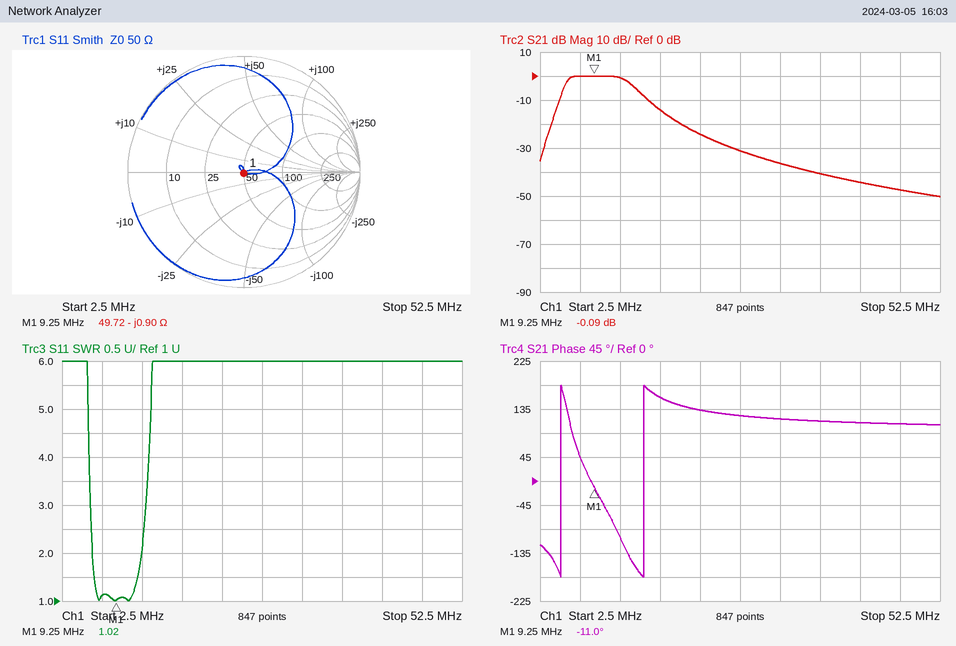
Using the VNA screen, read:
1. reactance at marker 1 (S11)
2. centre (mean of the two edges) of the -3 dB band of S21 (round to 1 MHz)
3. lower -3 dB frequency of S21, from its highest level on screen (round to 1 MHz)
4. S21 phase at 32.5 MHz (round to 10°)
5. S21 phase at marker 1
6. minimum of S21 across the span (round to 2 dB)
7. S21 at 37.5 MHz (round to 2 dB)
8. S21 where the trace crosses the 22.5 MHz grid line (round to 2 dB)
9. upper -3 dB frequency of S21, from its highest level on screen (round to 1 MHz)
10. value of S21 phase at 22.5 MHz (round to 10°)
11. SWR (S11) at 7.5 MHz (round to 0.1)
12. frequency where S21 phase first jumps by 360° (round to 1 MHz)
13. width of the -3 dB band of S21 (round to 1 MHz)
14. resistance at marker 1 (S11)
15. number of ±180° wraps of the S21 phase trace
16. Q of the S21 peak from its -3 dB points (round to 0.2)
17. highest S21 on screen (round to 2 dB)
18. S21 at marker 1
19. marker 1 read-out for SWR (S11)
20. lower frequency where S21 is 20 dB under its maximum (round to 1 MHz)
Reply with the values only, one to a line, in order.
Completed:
-0.90 Ω
10 MHz
6 MHz
120°
-11.0°
-50 dB
-40 dB
-24 dB
14 MHz
130°
1.1
5 MHz
8 MHz
49.72 Ω
2
1.2
0 dB
-0.09 dB
1.02
4 MHz
